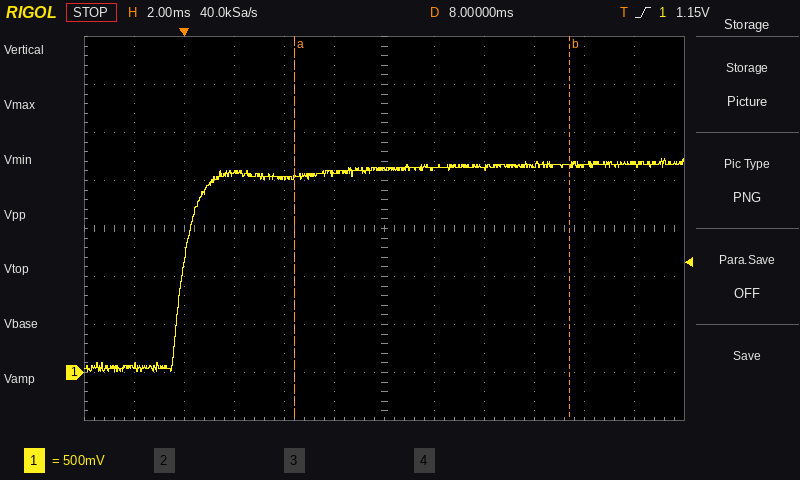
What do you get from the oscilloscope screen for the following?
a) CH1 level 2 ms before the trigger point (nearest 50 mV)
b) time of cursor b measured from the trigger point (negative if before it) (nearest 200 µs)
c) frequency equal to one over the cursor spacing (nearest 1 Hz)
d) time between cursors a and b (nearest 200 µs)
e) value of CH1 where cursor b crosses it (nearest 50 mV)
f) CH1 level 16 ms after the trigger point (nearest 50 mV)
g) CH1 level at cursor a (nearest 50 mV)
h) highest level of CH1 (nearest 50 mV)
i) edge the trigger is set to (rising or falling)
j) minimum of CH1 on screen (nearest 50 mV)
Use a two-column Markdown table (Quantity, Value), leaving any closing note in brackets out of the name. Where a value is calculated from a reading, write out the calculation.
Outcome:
| Quantity | Value |
|---|---|
| CH1 level 2 ms before the trigger point | 50 mV |
| time of cursor b measured from the trigger point (negative if before it) | +15.4 ms |
| frequency equal to one over the cursor spacing | 1 / 11.0 ms ≈ 91 Hz |
| time between cursors a and b | 11.0 ms |
| value of CH1 where cursor b crosses it | 2.15 V |
| CH1 level 16 ms after the trigger point | 2.15 V |
| CH1 level at cursor a | 2.05 V |
| highest level of CH1 | 2.25 V |
| edge the trigger is set to | rising |
| minimum of CH1 on screen | 0 mV |
